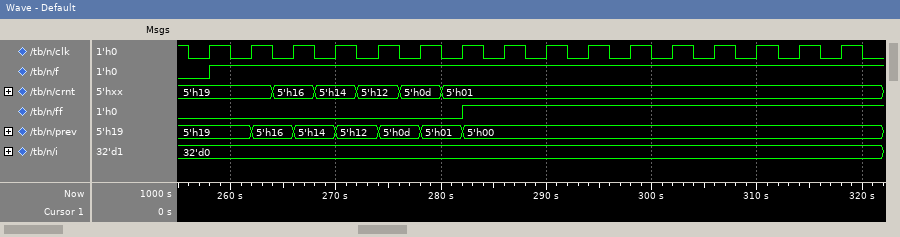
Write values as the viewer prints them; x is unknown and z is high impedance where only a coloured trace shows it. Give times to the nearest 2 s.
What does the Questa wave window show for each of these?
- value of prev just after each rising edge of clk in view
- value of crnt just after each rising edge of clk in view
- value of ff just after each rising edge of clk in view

5'h19, 5'h16, 5'h14, 5'h12, 5'h0d, 5'h01, 5'h00, 5'h00, 5'h00, 5'h00, 5'h00, 5'h00, 5'h00, 5'h00, 5'h00, 5'h00
5'h19, 5'h19, 5'h16, 5'h14, 5'h12, 5'h0d, 5'h01, 5'h01, 5'h01, 5'h01, 5'h01, 5'h01, 5'h01, 5'h01, 5'h01, 5'h01
0 0 0 0 0 0 1 1 1 1 1 1 1 1 1 1
